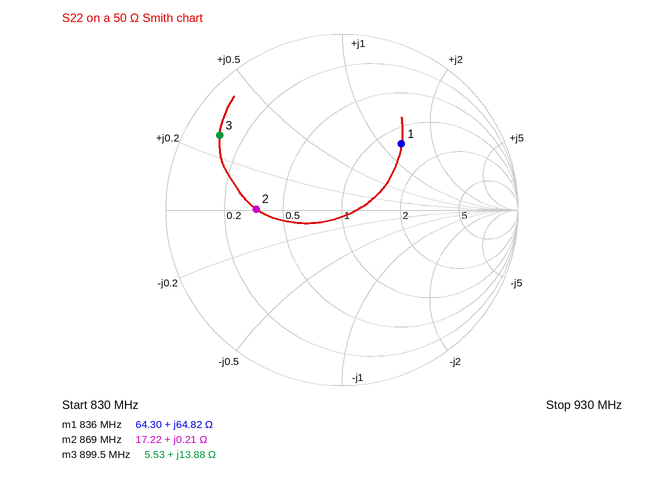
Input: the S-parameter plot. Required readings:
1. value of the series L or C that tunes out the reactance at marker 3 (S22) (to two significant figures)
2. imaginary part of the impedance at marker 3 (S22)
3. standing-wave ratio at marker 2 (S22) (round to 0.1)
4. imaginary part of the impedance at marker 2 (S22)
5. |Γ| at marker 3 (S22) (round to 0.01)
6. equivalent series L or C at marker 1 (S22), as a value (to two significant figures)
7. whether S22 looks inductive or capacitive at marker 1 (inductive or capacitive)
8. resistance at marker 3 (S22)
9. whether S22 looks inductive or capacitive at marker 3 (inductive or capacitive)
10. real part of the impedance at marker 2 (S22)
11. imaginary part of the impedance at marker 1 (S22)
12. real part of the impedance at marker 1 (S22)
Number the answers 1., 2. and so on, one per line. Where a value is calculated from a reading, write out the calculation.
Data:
1. C = 1/(2π × 899.5 MHz × 13.88 Ω) ≈ 13 pF
2. +13.88 Ω
3. 2.9
4. +0.21 Ω
5. 0.81
6. L = 64.82 Ω/(2π × 836 MHz) ≈ 12 nH
7. inductive
8. 5.53 Ω
9. inductive
10. 17.22 Ω
11. +64.82 Ω
12. 64.30 Ω
